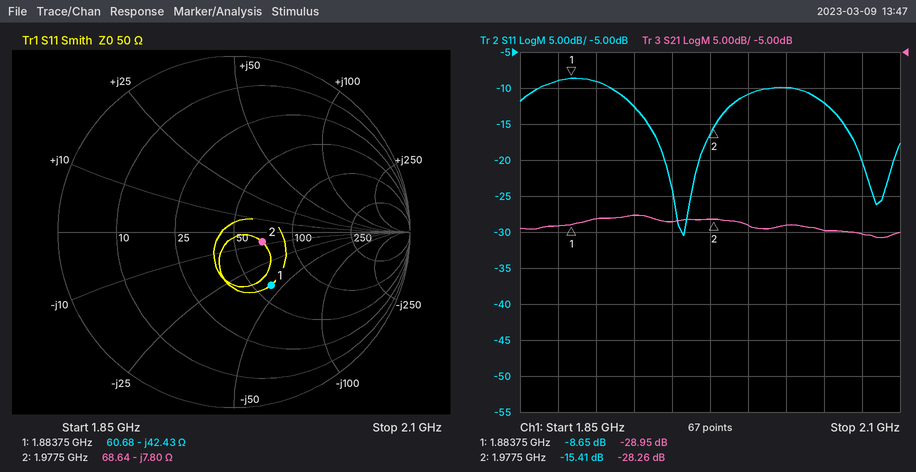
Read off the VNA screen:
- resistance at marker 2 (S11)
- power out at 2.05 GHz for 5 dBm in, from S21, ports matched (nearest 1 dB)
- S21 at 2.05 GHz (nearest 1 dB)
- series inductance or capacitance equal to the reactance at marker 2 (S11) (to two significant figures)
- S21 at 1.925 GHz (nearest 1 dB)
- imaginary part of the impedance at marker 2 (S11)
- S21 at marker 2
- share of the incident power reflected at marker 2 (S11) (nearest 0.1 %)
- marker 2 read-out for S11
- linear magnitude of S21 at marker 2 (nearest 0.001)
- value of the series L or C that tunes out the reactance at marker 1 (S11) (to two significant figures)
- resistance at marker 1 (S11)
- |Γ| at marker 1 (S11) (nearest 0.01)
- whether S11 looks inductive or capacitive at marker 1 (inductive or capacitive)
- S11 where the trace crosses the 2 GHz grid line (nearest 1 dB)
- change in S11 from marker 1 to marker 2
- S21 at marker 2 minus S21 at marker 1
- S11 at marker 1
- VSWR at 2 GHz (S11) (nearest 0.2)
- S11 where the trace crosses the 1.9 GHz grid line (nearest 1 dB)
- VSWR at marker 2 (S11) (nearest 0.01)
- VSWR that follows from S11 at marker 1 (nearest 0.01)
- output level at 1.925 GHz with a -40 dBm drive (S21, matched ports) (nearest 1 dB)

68.64 Ω
-25 dBm
-30 dB
10 pF
-28 dB
-7.80 Ω
-28.26 dB
2.9 %
-15.41 dB
0.039
3.6 nH
60.68 Ω
0.37
capacitive
-11 dB
-6.76 dB
0.69 dB
-8.65 dB
1.8
-9 dB
1.41
2.17
-68 dBm
